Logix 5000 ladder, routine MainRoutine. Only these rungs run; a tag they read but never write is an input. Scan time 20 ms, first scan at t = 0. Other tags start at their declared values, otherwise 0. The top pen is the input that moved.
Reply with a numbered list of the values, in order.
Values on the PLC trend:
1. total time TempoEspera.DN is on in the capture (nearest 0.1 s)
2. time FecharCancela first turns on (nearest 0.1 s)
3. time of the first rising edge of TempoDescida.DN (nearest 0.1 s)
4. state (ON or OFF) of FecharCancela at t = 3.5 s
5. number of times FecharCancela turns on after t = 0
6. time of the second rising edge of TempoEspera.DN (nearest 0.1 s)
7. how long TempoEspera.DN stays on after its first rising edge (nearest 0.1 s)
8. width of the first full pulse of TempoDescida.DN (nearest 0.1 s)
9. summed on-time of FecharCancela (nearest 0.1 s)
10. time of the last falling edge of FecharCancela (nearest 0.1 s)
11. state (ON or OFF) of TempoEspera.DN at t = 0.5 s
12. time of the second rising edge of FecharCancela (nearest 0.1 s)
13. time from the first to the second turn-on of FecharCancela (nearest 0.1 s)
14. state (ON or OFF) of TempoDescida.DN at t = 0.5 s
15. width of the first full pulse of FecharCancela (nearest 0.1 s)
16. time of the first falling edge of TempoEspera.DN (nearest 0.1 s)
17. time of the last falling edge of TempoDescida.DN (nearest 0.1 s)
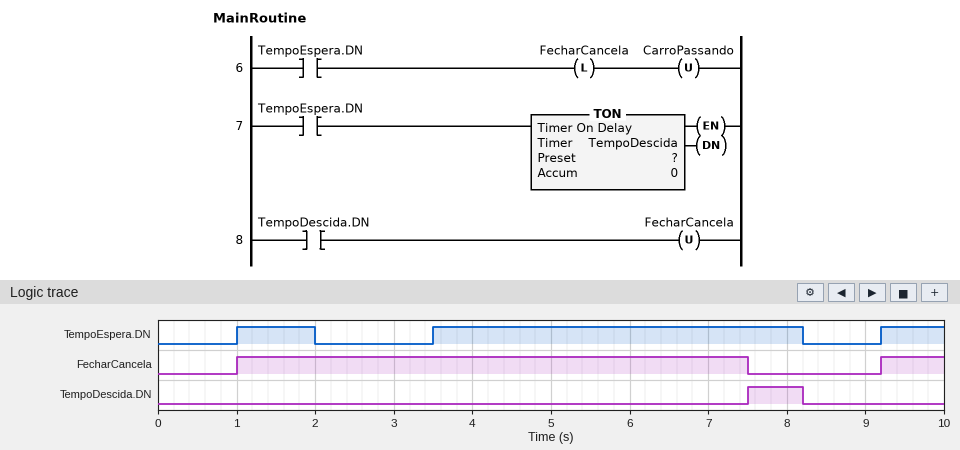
1. 6.5 s
2. 1.0 s
3. 7.5 s
4. ON
5. 2
6. 3.5 s
7. 1.0 s
8. 0.7 s
9. 7.3 s
10. 7.5 s
11. OFF
12. 9.2 s
13. 8.2 s
14. OFF
15. 6.5 s
16. 2.0 s
17. 8.2 s
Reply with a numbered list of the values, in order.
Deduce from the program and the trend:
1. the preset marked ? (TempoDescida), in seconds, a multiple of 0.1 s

1. 4.0 s
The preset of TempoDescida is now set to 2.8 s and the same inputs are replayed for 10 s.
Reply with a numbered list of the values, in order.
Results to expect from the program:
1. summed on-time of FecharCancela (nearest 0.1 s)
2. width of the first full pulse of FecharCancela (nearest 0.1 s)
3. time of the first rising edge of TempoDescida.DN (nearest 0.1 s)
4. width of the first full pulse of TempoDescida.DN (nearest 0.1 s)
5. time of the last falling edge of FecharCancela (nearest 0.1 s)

1. 6.1 s
2. 5.3 s
3. 6.3 s
4. 1.9 s
5. 6.3 s
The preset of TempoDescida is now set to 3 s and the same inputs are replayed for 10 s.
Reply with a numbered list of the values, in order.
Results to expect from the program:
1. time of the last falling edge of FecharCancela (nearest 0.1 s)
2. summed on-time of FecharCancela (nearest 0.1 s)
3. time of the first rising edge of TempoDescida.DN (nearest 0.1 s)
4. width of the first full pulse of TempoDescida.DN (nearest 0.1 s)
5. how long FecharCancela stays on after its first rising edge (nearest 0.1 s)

1. 6.5 s
2. 6.3 s
3. 6.5 s
4. 1.7 s
5. 5.5 s
